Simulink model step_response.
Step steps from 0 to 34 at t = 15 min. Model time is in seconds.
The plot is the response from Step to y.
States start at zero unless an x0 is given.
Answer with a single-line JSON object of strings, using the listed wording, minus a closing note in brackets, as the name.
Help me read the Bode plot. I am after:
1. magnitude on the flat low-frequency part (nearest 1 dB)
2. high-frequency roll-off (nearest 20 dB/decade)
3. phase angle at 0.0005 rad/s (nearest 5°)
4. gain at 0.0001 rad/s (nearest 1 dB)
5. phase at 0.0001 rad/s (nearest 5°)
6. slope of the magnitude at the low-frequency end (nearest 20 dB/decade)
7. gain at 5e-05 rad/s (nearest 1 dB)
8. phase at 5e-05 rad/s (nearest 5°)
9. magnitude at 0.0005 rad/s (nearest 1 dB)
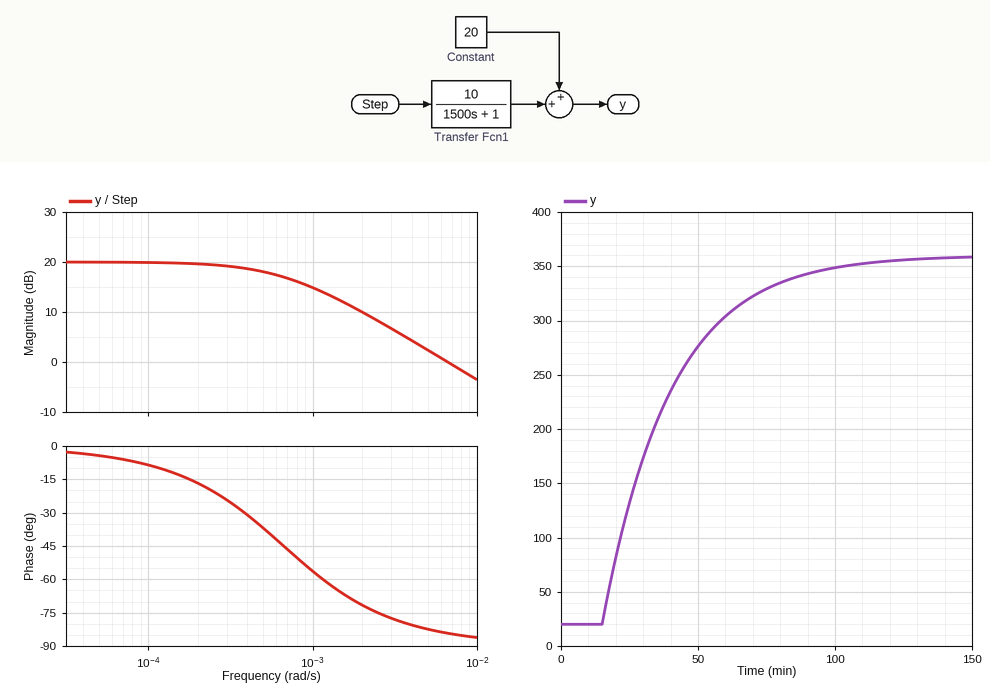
{"magnitude on the flat low-frequency part": "20 dB", "high-frequency roll-off": "-20 dB/decade", "phase angle at 0.0005 rad/s": "-35°", "gain at 0.0001 rad/s": "20 dB", "phase at 0.0001 rad/s": "-10°", "slope of the magnitude at the low-frequency end": "0 dB/decade", "gain at 5e-05 rad/s": "20 dB", "phase at 5e-05 rad/s": "-5°", "magnitude at 0.0005 rad/s": "18 dB"}
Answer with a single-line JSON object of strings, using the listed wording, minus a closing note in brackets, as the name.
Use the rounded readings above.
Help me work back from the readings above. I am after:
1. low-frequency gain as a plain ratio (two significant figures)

{"low-frequency gain as a plain ratio": "10"}
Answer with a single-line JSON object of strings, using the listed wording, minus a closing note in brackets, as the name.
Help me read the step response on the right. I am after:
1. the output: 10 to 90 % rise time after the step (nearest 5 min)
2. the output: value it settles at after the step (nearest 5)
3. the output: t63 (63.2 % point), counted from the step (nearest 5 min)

{"the output: 10 to 90 % rise time after the step": "55 min", "the output: value it settles at after the step": "360", "the output: t63 (63.2 % point), counted from the step": "25 min"}
